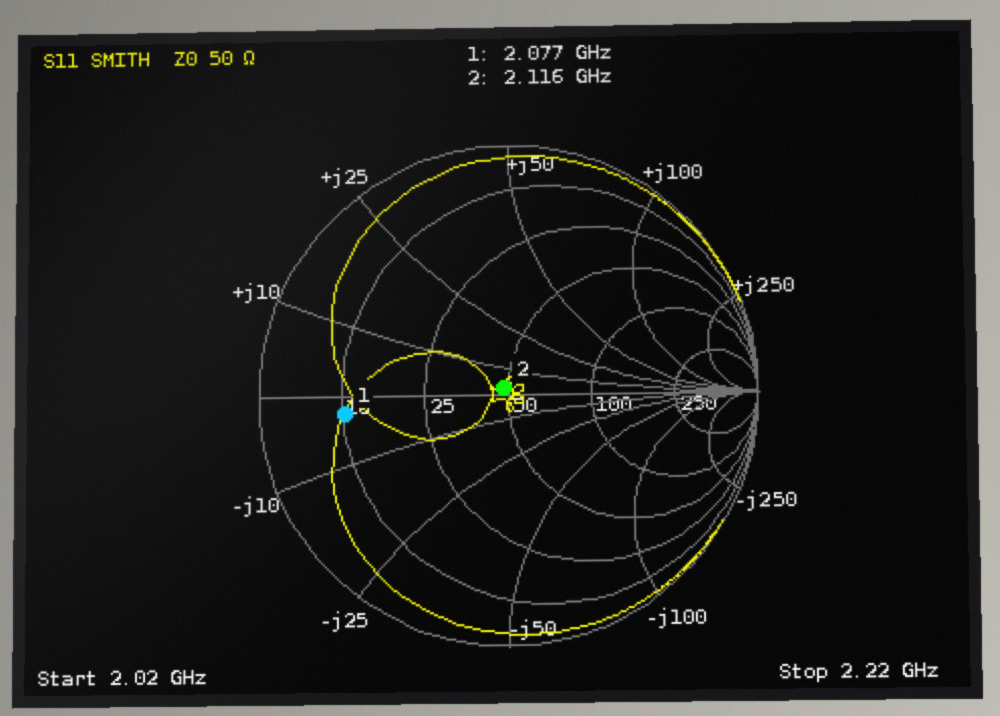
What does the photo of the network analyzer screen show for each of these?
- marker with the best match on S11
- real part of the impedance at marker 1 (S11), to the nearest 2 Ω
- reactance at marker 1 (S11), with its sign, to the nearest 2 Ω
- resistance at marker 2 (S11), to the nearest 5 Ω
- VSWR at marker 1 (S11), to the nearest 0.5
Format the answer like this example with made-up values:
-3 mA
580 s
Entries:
marker 2
10 Ω
-2 Ω
50 Ω
5.0
